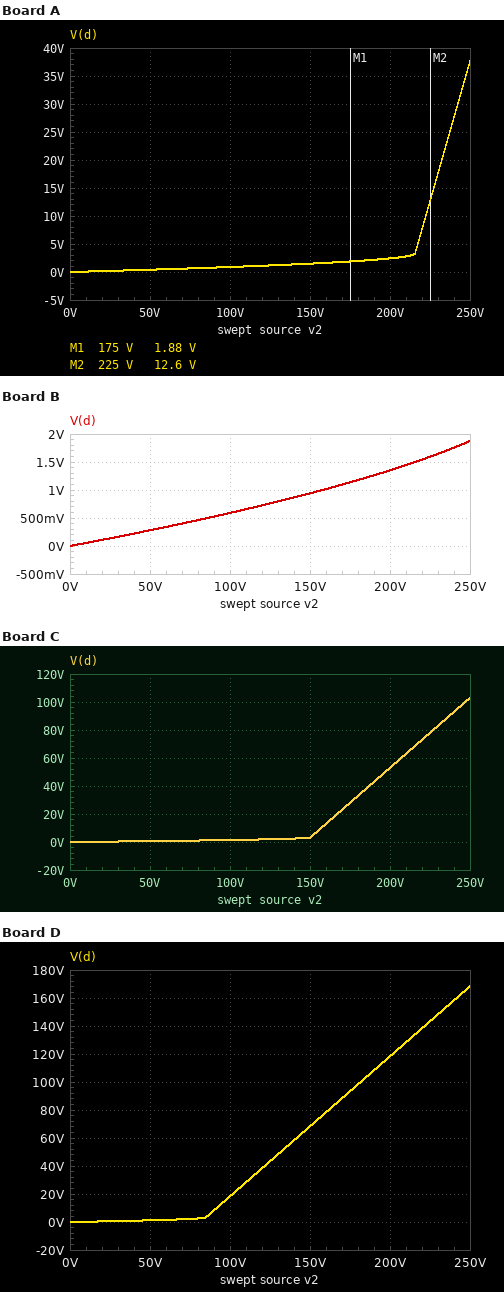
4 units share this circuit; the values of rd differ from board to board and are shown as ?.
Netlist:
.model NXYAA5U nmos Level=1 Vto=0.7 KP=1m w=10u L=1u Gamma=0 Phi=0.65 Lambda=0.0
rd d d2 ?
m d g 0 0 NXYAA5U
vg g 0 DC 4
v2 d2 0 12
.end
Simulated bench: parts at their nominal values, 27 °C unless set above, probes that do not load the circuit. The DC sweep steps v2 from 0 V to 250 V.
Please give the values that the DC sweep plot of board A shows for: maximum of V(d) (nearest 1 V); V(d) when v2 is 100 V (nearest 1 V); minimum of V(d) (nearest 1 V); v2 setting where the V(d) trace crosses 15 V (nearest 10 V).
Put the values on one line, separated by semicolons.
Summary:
38 V; 1 V; 0 V; 230 V
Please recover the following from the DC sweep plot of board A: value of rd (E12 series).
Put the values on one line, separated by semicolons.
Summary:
3.9 kΩ
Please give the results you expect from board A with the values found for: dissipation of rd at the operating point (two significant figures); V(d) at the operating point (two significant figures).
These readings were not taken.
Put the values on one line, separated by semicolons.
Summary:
36 mW; 94 mV
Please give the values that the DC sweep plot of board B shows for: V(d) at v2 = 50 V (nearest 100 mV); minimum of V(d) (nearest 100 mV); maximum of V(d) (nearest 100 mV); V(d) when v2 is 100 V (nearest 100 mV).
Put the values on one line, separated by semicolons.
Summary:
300 mV; 0 V; 1.9 V; 600 mV
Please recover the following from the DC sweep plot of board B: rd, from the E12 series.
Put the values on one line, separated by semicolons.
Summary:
5.6 kΩ
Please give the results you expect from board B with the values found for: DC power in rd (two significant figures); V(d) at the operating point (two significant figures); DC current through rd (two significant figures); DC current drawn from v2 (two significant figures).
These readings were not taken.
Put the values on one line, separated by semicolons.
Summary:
25 mW; 65 mV; 2.1 mA; 2.1 mA
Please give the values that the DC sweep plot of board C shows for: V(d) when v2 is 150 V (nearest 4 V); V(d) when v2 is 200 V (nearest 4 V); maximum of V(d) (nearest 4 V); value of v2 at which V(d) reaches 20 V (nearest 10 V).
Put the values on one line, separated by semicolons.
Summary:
4 V; 52 V; 104 V; 170 V
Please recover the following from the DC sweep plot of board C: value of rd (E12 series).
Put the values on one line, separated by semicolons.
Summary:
2.7 kΩ
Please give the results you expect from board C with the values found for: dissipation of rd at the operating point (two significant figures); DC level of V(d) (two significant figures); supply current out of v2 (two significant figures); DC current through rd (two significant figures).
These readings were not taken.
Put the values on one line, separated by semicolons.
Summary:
52 mW; 140 mV; 4.4 mA; 4.4 mA
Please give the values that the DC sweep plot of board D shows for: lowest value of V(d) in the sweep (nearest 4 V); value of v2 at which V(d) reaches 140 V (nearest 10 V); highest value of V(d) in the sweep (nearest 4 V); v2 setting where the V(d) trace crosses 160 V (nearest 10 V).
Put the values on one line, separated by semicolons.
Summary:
0 V; 220 V; 168 V; 240 V
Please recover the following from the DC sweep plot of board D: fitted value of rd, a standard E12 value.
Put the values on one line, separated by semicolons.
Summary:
1.5 kΩ
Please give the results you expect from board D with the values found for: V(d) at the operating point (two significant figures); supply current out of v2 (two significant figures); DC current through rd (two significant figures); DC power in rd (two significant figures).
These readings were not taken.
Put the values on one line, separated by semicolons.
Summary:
250 mV; 7.8 mA; 7.8 mA; 92 mW
